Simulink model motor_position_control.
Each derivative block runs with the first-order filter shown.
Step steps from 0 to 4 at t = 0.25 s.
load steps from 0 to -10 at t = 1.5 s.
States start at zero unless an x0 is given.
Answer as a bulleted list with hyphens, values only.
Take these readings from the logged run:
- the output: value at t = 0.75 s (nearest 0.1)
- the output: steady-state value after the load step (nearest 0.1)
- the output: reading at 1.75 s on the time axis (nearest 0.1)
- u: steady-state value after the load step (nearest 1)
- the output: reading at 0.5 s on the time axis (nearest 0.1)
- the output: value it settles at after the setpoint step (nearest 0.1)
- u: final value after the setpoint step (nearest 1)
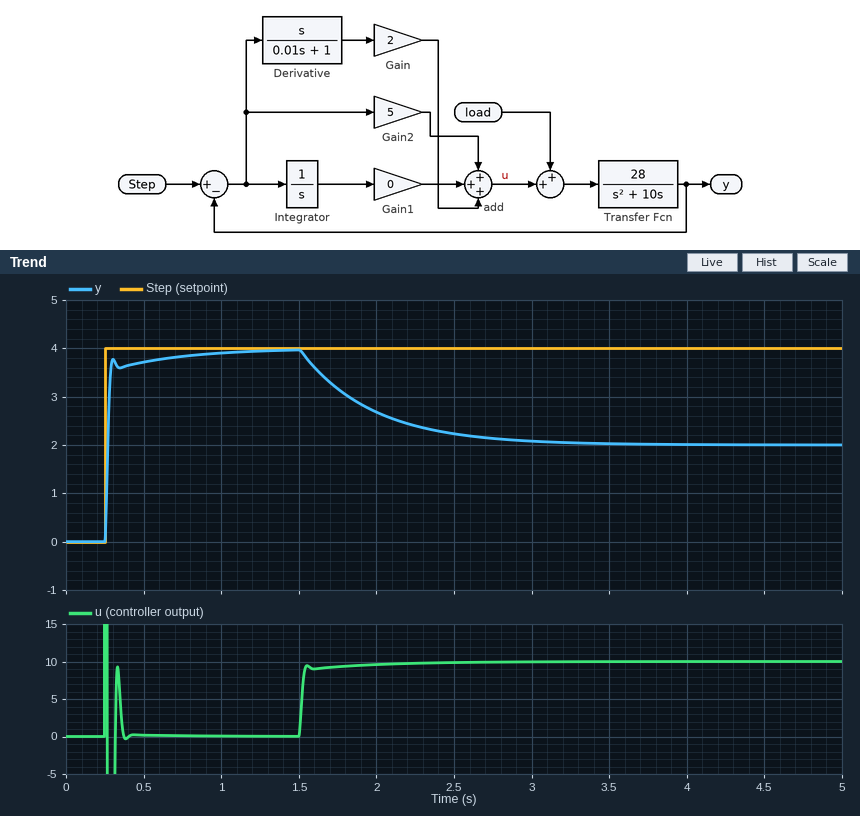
- 3.8
- 2.0
- 3.2
- 10
- 3.7
- 4.0
- 0
